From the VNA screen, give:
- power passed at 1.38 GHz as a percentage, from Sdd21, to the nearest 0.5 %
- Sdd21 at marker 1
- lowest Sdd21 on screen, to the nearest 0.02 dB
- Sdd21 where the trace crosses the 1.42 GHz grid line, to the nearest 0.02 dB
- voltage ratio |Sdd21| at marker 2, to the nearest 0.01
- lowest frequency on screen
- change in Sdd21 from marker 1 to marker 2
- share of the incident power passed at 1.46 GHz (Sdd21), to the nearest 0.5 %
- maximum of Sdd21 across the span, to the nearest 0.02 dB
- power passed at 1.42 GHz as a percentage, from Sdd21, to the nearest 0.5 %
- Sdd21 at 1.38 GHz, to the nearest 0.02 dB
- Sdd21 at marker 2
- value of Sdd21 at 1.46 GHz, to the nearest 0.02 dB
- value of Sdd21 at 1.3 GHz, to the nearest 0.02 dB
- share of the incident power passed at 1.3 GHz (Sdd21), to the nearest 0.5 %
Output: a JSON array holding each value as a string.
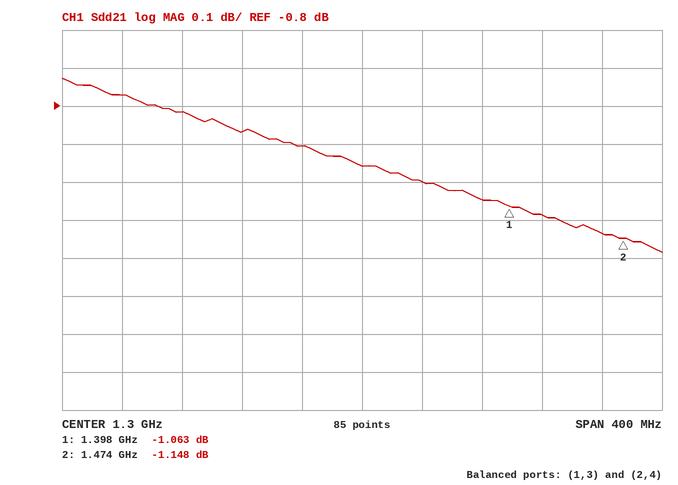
["78.5 %", "-1.063 dB", "-1.18 dB", "-1.08 dB", "0.88", "1.1 GHz", "-0.085 dB", "77.0 %", "-0.72 dB", "78.0 %", "-1.04 dB", "-1.148 dB", "-1.14 dB", "-0.96 dB", "80.0 %"]
